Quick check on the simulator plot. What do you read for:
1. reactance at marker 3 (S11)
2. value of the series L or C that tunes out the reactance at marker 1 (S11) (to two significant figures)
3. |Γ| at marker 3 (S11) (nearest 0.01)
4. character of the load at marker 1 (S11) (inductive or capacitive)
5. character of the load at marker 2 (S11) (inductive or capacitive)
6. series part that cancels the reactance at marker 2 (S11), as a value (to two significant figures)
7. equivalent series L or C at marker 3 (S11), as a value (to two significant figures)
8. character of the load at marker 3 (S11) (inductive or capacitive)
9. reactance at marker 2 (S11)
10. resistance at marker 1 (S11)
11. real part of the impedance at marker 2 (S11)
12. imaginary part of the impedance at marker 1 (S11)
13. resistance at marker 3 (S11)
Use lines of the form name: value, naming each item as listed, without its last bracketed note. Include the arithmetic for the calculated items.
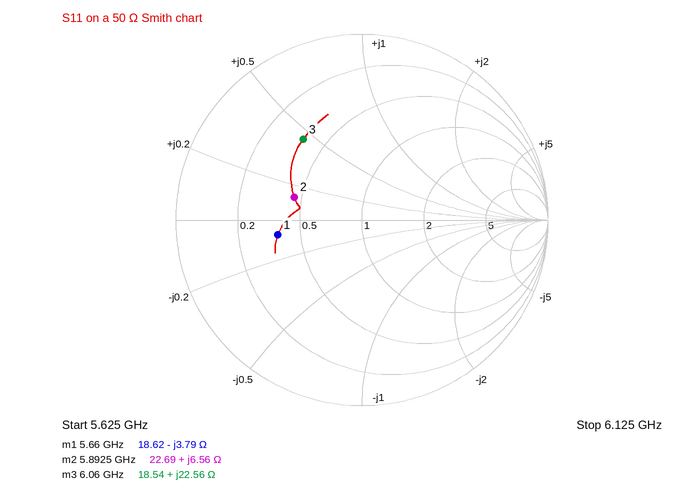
reactance at marker 3: +22.56 Ω
value of the series L or C that tunes out the reactance at marker 1 (S11): L = 3.79 Ω/(2π × 5.66 GHz) ≈ 107 pH, so 110 pH to two significant figures
|Γ| at marker 3 (S11): 0.54
character of the load at marker 1 (S11): capacitive
character of the load at marker 2 (S11): inductive
series part that cancels the reactance at marker 2 (S11), as a value: C = 1/(2π × 5.8925 GHz × 6.56 Ω) ≈ 4.1 pF
equivalent series L or C at marker 3 (S11), as a value: L = 22.56 Ω/(2π × 6.06 GHz) ≈ 592 pH, so 590 pH to two significant figures
character of the load at marker 3 (S11): inductive
reactance at marker 2: +6.56 Ω
resistance at marker 1: 18.62 Ω
real part of the impedance at marker 2: 22.69 Ω
imaginary part of the impedance at marker 1: -3.79 Ω
resistance at marker 3: 18.54 Ω
